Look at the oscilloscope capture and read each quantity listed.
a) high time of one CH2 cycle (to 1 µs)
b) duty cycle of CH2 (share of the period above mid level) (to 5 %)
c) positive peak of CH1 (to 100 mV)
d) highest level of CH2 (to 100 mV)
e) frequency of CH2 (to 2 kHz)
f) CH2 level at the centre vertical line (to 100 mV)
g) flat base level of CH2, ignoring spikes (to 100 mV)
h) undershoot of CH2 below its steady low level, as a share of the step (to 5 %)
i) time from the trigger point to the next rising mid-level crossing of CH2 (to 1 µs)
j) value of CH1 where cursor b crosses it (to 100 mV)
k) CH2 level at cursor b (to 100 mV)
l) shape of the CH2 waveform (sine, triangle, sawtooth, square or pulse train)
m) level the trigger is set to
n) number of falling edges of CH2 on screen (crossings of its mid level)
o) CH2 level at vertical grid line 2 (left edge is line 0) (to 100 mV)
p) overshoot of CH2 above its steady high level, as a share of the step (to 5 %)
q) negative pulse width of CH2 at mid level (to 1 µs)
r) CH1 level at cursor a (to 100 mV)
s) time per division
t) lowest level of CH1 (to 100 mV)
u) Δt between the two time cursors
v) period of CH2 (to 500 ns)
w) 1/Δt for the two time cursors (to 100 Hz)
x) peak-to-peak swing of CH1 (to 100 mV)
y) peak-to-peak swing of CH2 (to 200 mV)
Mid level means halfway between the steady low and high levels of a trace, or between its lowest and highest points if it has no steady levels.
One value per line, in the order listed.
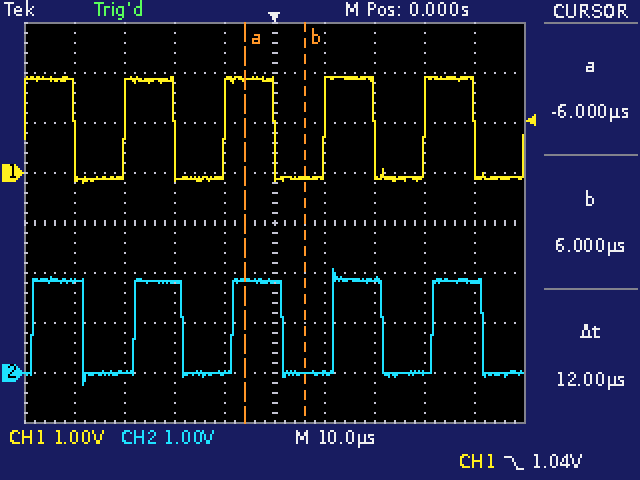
10 µs
50 %
1.9 V
2.1 V
50 kHz
1.8 V
0.0 V
15 %
12 µs
-100 mV
0.0 V
square
1.04 V
5
0.0 V
15 %
10 µs
1.9 V
10 µs
-200 mV
12 µs
20.0 µs
83.3 kHz
2.1 V
2.4 V
